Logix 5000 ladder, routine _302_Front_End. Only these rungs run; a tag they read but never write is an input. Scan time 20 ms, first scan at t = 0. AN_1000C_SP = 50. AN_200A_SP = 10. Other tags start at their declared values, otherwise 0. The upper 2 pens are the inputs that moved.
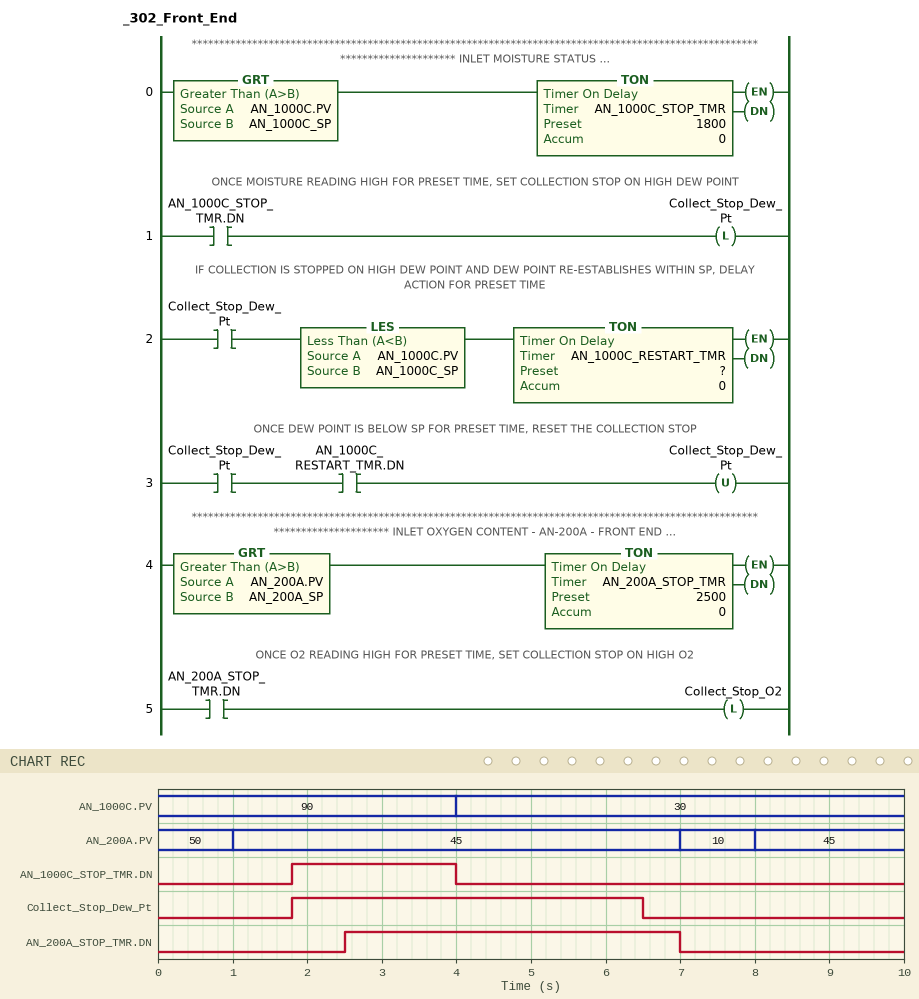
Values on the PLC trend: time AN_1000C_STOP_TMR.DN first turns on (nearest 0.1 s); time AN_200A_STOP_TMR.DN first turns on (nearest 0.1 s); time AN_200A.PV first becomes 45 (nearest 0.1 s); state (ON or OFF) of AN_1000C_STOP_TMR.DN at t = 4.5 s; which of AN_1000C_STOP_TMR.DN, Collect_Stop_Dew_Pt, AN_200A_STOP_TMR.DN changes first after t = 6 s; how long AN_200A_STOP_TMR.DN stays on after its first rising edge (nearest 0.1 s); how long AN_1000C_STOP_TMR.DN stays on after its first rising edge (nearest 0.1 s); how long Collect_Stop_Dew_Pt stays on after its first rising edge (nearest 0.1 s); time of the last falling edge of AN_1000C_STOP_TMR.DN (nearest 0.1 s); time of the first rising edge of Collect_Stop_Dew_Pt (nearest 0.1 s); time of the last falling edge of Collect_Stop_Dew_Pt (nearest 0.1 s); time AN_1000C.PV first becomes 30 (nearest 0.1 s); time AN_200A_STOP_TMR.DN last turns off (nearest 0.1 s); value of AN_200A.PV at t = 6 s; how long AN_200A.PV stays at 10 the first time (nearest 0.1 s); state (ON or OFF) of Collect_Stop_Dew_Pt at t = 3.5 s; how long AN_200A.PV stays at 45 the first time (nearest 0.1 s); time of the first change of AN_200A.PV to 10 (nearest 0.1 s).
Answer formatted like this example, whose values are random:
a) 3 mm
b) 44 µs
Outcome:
a) 1.8 s
b) 2.5 s
c) 1.0 s
d) OFF
e) Collect_Stop_Dew_Pt
f) 4.5 s
g) 2.2 s
h) 4.7 s
i) 4.0 s
j) 1.8 s
k) 6.5 s
l) 4.0 s
m) 7.0 s
n) 45
o) 1.0 s
p) ON
q) 6.0 s
r) 7.0 s
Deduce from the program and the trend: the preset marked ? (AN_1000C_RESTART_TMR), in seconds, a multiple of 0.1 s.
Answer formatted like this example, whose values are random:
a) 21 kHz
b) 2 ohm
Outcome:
a) 2.5 s
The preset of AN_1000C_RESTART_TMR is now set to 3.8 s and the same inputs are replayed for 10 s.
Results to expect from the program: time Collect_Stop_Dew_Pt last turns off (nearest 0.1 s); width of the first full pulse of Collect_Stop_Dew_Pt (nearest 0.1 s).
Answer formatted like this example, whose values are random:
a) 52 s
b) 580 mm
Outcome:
a) 7.8 s
b) 6.0 s
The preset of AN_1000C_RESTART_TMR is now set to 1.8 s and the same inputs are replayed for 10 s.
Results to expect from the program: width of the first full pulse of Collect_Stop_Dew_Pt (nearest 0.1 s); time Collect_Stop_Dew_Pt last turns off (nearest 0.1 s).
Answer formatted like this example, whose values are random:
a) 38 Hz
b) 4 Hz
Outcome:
a) 4.0 s
b) 5.8 s
